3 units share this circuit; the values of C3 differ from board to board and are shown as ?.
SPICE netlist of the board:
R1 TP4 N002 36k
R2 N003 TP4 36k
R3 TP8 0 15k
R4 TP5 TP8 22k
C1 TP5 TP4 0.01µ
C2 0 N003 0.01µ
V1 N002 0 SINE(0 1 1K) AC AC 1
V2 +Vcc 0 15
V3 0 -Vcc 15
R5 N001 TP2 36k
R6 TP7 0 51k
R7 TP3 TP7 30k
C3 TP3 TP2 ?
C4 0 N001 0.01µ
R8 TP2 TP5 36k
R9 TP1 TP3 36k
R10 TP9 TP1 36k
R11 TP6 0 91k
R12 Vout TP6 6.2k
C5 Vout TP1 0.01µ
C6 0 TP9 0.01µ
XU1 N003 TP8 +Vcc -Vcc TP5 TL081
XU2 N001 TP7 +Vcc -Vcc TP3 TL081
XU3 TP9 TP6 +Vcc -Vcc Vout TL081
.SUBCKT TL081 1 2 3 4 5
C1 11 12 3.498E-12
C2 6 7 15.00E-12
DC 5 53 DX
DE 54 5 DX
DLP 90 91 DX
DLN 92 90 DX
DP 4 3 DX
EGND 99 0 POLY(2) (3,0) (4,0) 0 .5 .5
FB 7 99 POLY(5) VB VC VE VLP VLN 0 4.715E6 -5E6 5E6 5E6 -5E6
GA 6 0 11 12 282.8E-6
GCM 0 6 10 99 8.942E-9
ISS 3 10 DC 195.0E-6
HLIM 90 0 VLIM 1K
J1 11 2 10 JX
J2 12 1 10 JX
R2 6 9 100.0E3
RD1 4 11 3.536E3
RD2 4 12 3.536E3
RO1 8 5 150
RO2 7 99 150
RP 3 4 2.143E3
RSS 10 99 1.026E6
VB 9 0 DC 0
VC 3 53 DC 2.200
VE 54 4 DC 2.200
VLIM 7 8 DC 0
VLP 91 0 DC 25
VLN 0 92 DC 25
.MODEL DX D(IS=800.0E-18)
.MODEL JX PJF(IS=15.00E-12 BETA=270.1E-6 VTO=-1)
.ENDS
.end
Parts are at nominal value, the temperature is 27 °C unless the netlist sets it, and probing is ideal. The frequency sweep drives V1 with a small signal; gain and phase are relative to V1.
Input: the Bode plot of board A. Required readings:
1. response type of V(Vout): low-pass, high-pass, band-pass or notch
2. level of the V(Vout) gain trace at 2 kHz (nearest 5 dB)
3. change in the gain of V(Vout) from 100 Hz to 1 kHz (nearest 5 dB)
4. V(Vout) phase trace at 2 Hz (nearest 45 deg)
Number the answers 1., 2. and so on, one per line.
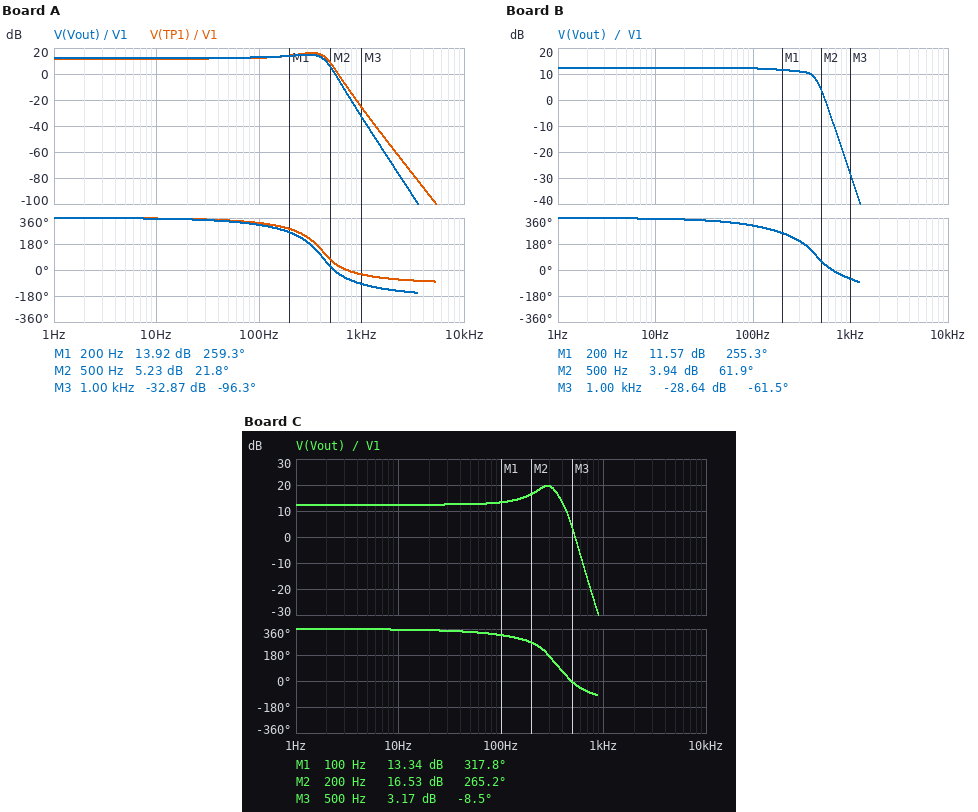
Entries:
1. low-pass
2. -70 dB
3. -45 dB
4. 360 deg
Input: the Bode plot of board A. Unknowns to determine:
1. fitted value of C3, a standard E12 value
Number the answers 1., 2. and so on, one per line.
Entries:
1. 15 nF
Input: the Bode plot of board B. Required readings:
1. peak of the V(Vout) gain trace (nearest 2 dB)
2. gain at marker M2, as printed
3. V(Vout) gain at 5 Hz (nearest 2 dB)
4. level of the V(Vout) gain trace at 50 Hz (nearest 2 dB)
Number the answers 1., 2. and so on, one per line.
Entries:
1. 12 dB
2. 3.94 dB
3. 12 dB
4. 12 dB
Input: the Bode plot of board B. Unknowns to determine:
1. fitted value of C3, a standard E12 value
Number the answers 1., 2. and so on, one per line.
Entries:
1. 6.8 nF
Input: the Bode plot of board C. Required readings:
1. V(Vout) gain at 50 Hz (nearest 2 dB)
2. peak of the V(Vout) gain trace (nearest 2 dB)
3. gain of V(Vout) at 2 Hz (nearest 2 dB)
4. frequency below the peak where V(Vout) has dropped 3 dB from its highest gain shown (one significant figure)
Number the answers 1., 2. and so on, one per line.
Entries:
1. 12 dB
2. 20 dB
3. 12 dB
4. 200 Hz
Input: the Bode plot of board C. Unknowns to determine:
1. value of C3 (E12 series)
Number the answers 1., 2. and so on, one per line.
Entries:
1. 22 nF
